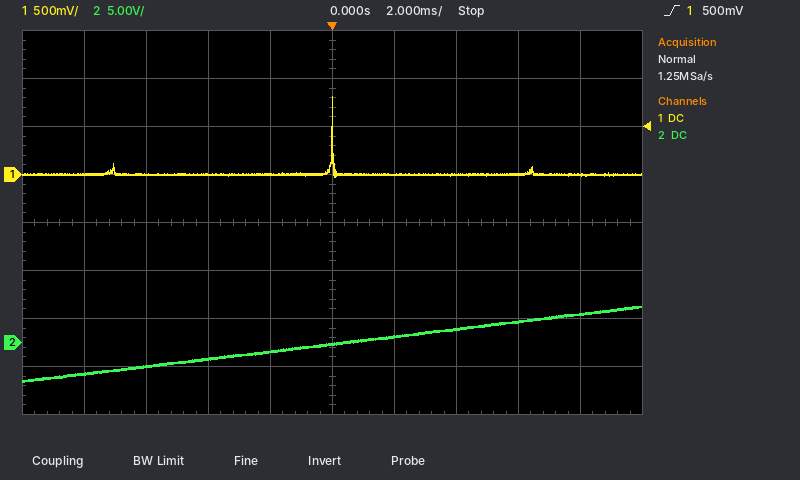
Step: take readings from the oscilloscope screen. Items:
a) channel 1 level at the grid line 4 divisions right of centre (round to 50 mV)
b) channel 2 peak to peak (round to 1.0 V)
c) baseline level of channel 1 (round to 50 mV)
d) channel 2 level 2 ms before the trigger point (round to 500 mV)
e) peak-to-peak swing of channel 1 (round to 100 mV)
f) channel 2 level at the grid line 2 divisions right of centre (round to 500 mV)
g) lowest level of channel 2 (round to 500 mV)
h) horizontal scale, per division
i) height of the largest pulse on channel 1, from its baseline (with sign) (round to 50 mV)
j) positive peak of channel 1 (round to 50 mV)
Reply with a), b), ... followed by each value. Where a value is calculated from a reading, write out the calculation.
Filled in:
a) 0 mV
b) 8.0 V
c) 0 mV
d) -1.0 V
e) 800 mV
f) 1.5 V
g) -4.0 V
h) 2 ms
i) 800 mV − (0 mV) = +800 mV
j) 800 mV
